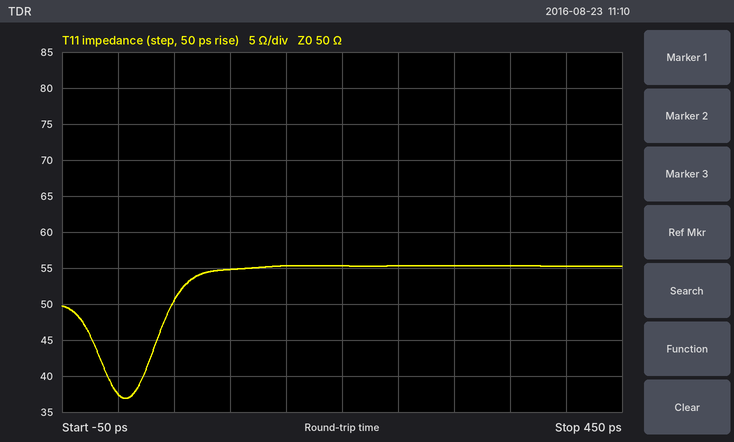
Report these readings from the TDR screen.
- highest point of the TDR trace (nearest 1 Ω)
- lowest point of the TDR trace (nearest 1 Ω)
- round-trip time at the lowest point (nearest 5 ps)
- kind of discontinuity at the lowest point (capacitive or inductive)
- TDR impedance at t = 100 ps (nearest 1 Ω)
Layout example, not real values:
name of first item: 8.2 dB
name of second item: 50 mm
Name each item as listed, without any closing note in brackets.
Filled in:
highest point of the TDR trace: 55 Ω
lowest point of the TDR trace: 37 Ω
round-trip time at the lowest point: 5 ps
kind of discontinuity at the lowest point: capacitive
TDR impedance at t = 100 ps: 55 Ω
